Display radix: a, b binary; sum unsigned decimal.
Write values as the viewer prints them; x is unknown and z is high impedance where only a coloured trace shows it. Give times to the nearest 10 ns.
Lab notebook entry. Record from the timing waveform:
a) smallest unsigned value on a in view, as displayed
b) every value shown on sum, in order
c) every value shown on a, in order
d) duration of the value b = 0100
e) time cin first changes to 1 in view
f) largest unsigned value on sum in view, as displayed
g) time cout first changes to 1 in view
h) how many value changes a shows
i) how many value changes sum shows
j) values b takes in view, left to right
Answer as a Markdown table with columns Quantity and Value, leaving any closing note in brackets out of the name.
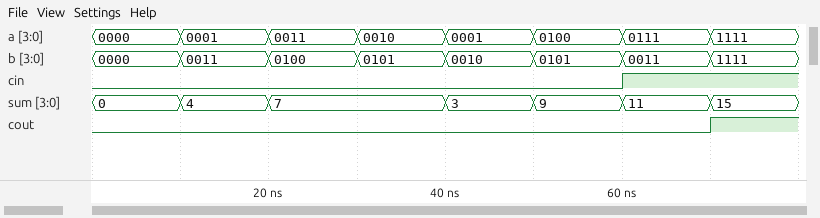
| Quantity | Value |
|---|---|
| smallest unsigned value on a in view, as displayed | 0000 |
| every value shown on sum, in order | 0, 4, 7, 3, 9, 11, 15 |
| every value shown on a, in order | 0000, 0001, 0011, 0010, 0001, 0100, 0111, 1111 |
| duration of the value b = 0100 | 10 ns |
| time cin first changes to 1 in view | 60 ns |
| largest unsigned value on sum in view, as displayed | 15 |
| time cout first changes to 1 in view | 70 ns |
| how many value changes a shows | 7 |
| how many value changes sum shows | 6 |
| values b takes in view, left to right | 0000, 0011, 0100, 0101, 0010, 0101, 0011, 1111 |
